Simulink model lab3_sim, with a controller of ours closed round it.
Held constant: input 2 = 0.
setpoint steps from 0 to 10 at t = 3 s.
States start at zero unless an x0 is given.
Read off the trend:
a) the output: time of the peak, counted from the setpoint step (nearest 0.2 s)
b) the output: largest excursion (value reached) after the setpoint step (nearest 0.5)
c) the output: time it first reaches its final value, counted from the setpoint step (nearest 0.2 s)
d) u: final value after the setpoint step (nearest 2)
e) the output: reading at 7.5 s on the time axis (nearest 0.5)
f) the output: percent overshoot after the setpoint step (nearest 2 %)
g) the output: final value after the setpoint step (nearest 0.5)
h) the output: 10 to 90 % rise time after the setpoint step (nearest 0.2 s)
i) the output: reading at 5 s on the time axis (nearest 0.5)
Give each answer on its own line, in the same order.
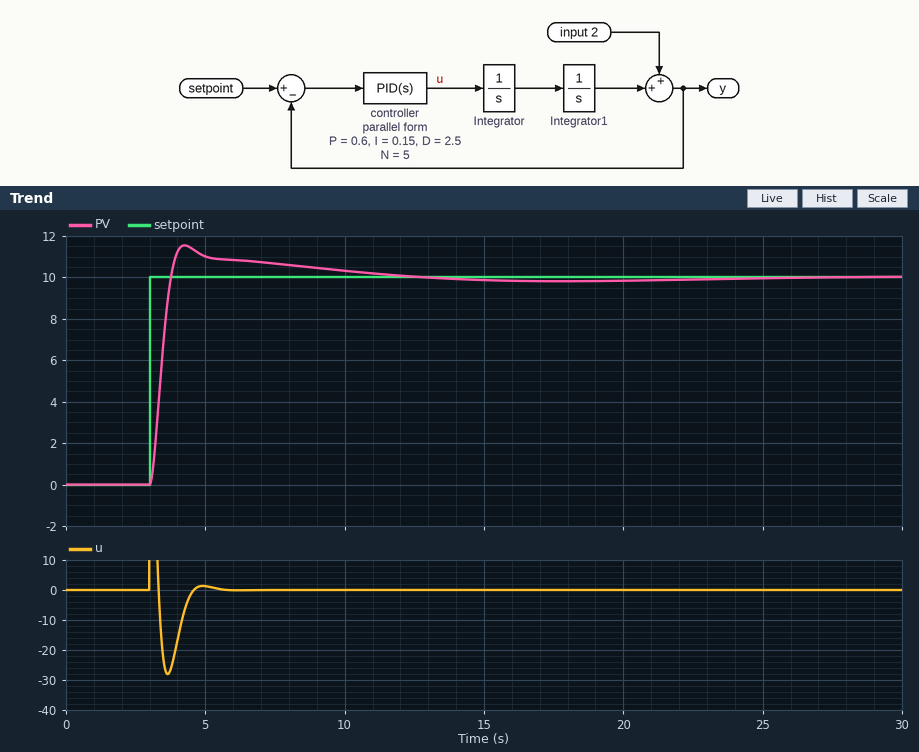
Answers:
1.2 s
11.5
0.8 s
0
10.5
16 %
10.0
0.6 s
11.0
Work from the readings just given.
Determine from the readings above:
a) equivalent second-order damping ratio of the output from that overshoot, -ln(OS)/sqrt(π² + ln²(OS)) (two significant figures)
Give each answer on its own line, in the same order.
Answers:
0.50
